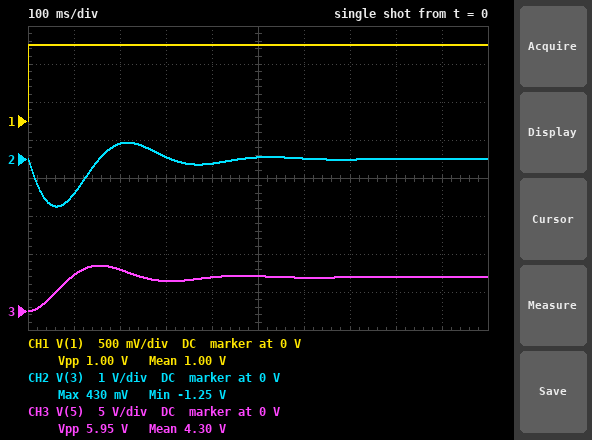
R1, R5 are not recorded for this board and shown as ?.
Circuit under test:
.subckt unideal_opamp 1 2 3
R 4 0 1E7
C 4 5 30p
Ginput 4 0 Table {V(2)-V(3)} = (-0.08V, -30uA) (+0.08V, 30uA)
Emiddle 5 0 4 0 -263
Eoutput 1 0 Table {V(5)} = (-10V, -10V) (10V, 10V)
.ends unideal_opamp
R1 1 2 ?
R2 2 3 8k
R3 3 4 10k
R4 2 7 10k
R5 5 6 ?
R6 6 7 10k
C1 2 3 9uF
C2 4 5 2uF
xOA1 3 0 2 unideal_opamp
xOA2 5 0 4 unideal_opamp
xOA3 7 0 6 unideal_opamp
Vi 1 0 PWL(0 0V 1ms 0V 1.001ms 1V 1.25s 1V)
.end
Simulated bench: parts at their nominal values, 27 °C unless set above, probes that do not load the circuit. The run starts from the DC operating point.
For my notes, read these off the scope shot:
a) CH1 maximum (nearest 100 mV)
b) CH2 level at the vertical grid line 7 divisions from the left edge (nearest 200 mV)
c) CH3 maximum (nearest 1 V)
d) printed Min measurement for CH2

1.0 V
0 V
6 V
-1.25 V
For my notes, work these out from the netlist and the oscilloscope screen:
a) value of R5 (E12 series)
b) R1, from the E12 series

12 kΩ
2.7 kΩ
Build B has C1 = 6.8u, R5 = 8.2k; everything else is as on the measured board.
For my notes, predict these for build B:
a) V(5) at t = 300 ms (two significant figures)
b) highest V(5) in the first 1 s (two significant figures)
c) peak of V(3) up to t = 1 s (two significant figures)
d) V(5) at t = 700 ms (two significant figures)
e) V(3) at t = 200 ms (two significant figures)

3.1 V
4.1 V
440 mV
3.0 V
180 mV
